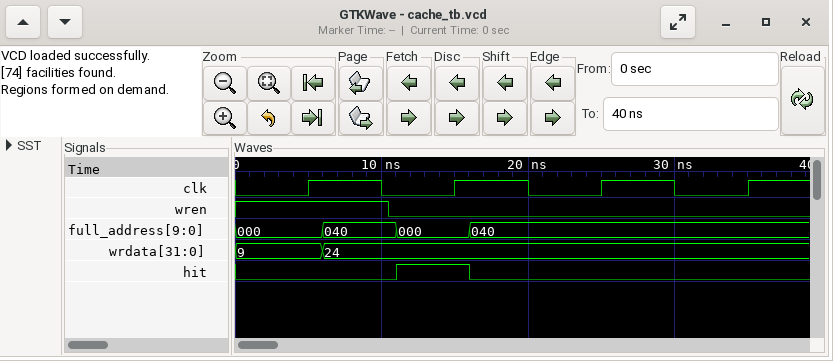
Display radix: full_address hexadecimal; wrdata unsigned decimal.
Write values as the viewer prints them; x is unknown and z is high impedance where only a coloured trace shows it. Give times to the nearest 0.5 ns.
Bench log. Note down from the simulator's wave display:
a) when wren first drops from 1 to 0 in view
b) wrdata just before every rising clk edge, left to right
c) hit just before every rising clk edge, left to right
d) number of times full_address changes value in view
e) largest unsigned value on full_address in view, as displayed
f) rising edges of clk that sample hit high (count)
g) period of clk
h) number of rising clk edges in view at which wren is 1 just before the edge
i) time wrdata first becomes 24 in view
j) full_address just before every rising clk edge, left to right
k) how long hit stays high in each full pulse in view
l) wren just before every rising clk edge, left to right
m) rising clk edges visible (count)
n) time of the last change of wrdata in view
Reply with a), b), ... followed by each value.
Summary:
a) 10.5 ns
b) 9, 24, 24, 24
c) 0 1 0 0
d) 3
e) 040
f) 1
g) 10 ns
h) 1
i) 6 ns
j) 000, 000, 040, 040
k) 5 ns
l) 1 0 0 0
m) 4
n) 6 ns
